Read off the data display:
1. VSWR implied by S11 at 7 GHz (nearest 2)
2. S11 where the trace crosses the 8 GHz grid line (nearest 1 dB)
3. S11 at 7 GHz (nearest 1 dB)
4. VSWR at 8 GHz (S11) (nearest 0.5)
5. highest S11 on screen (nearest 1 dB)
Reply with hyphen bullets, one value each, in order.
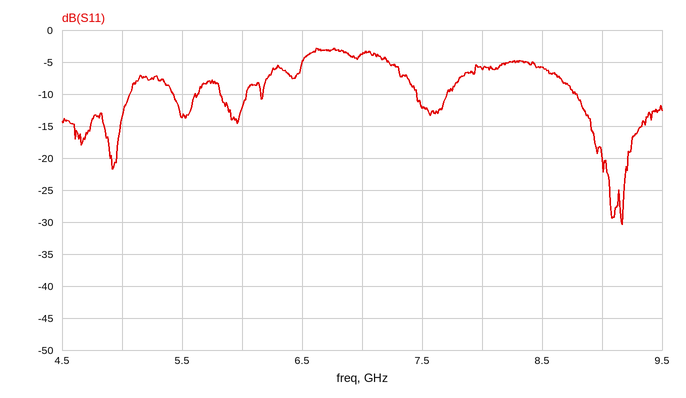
- 4
- -6 dB
- -4 dB
- 3.0
- -3 dB
